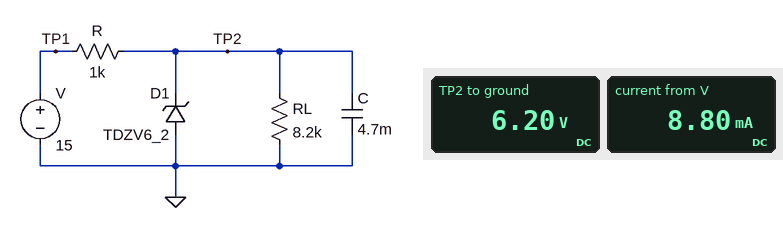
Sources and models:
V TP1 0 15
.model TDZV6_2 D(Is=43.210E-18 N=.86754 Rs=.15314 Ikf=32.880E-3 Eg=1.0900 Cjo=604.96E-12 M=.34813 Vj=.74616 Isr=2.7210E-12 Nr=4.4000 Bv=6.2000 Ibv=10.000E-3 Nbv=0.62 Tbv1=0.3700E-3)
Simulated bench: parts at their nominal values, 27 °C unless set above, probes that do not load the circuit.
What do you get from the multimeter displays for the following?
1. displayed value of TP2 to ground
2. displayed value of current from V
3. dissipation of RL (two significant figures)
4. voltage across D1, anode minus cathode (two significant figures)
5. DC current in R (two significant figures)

6.20 V
8.80 mA
4.7 mW
-6.2 V
8.8 mA
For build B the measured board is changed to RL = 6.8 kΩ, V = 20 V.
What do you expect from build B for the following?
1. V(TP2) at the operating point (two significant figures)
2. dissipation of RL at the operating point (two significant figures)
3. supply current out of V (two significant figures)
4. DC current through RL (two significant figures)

6.2 V
5.7 mW
14 mA
910 µA
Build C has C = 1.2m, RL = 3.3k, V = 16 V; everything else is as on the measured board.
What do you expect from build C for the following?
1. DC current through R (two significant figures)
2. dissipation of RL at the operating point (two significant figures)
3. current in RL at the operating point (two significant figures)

9.8 mA
12 mW
1.9 mA
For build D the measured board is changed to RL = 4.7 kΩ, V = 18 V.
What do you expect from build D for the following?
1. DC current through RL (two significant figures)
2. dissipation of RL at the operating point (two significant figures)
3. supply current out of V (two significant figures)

1.3 mA
8.2 mW
12 mA
